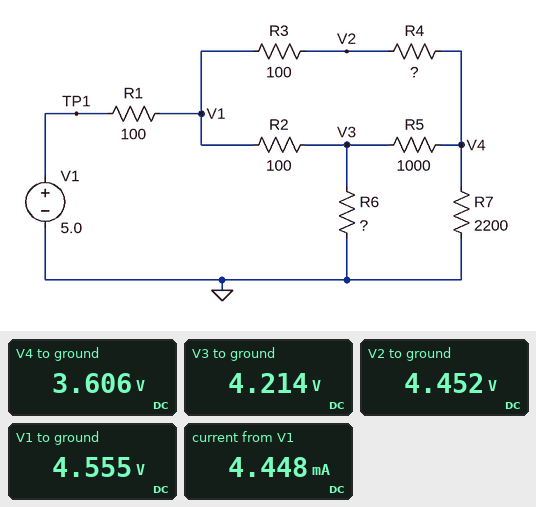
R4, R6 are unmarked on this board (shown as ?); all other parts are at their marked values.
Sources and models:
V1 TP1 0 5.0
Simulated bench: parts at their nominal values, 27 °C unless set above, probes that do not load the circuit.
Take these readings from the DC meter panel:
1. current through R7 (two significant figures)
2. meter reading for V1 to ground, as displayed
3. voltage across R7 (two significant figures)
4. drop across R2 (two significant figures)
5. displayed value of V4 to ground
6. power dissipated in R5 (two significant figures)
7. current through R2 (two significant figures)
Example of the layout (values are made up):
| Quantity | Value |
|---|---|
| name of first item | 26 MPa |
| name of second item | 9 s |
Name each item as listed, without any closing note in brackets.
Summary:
| Quantity | Value |
|---|---|
| current through R7 | 1.6 mA |
| meter reading for V1 to ground, as displayed | 4.555 V |
| voltage across R7 | 3.6 V |
| drop across R2 | 340 mV |
| displayed value of V4 to ground | 3.606 V |
| power dissipated in R5 | 370 µW |
| current through R2 | 3.4 mA |
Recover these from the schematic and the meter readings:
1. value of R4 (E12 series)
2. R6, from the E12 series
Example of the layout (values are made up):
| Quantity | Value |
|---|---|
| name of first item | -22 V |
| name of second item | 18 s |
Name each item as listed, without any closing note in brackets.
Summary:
| Quantity | Value |
|---|---|
| value of R4 | 820 Ω |
| R6, from the E12 series | 1.5 kΩ |
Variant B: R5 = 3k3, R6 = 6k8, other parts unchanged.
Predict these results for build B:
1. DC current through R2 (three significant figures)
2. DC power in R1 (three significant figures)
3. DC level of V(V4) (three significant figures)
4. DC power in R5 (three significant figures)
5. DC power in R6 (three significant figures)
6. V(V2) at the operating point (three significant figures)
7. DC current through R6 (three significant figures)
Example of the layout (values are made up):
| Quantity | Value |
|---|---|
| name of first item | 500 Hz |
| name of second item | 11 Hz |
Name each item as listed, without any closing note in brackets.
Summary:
| Quantity | Value |
|---|---|
| DC current through R2 | 1.02 mA |
| DC power in R1 | 535 µW |
| DC level of V(V4) | 3.58 V |
| DC power in R5 | 360 µW |
| DC power in R6 | 3.20 mW |
| V(V2) at the operating point | 4.64 V |
| DC current through R6 | 686 µA |
